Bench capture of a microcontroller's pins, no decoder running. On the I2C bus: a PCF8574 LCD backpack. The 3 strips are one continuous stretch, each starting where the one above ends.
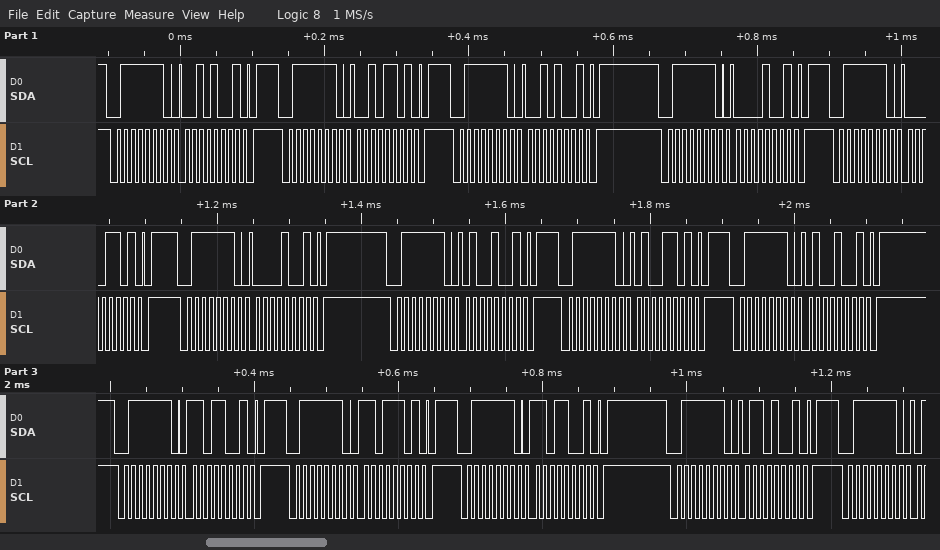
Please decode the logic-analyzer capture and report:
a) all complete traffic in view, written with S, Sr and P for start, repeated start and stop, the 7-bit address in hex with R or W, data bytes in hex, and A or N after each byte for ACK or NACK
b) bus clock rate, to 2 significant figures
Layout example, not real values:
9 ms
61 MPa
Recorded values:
S 3FW A 29 A P S 3FW A 2D A P S 3FW A 29 A P S 3FW A 09 A P S 3FW A 0D A P S 3FW A 09 A P S 3FW A 49 A P S 3FW A 4D A P S 3FW A 49 A P S 3FW A D9 A P S 3FW A DD A P S 3FW A D9 A P S 3FW A 69 A P S 3FW A
100 kHz
